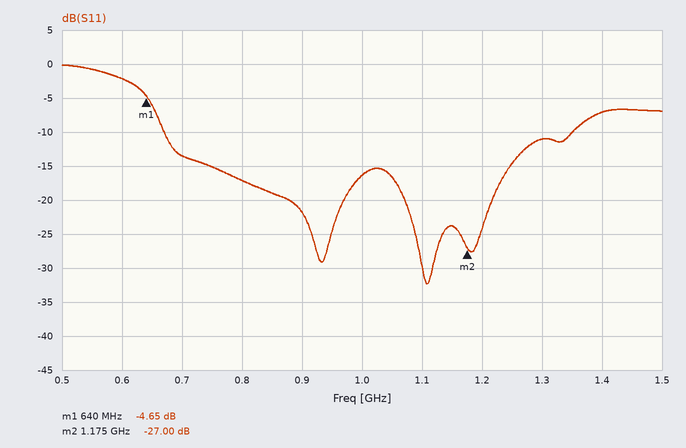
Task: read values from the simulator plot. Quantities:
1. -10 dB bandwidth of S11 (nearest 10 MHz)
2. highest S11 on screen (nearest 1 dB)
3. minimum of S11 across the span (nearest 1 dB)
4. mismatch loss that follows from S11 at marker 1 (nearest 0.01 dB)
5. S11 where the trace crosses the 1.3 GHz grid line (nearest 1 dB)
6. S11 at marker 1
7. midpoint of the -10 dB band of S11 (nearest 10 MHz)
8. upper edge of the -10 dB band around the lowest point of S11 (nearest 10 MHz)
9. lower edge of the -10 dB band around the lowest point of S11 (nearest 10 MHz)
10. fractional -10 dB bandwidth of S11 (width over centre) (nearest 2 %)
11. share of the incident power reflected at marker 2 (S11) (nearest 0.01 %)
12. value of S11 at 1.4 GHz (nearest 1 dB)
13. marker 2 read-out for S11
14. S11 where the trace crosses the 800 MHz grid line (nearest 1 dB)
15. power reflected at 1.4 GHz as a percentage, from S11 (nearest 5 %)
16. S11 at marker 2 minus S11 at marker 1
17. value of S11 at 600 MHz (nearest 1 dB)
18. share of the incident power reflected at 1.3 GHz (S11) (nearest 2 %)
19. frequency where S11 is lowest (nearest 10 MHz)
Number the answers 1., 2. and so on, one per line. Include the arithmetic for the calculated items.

1. 1.35 GHz − 670 MHz = 680 MHz
2. 0 dB
3. -32 dB
4. −10 log10(1 − 10^(-4.65/10)) ≈ 1.82 dB
5. -11 dB
6. -4.65 dB
7. 1.01 GHz
8. 1.35 GHz
9. 670 MHz
10. 680 MHz / 1.01 GHz ≈ 67.3 %, so 68 % to the nearest 2 %
11. 10^(-27/10) ≈ 0.20 %
12. -7 dB
13. -27.00 dB
14. -17 dB
15. 10^(-7/10) ≈ 20 %
16. -27 − (-4.65) = -22.35 dB
17. -2 dB
18. 10^(-11/10) ≈ 8 %
19. 1.11 GHz
